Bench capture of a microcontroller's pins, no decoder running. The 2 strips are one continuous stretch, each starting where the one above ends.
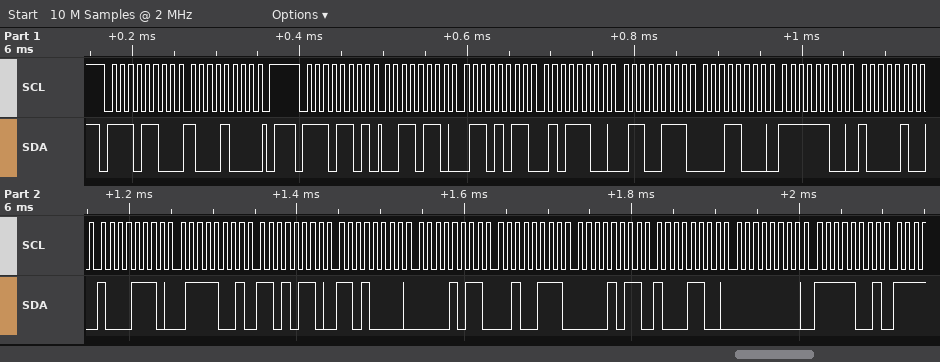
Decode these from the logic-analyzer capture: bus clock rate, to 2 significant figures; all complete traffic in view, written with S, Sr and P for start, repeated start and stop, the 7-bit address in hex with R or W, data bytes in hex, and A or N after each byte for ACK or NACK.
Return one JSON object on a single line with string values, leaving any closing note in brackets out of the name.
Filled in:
{"bus clock rate, to 2 significant figures": "100 kHz", "all complete traffic in view, written with S, Sr and P for start, repeated start and stop, the 7-bit address in hex with R or W, data bytes in hex, and A or N after each byte for ACK or NACK": "S 76W A 88 A P S 76R A 36 A 6B A 5C A 67 A 18 A FC A 84 A 8E A 79 A D6 A D0 A 0B A 27 A 0B A 8C A 00 A F9 A"}
